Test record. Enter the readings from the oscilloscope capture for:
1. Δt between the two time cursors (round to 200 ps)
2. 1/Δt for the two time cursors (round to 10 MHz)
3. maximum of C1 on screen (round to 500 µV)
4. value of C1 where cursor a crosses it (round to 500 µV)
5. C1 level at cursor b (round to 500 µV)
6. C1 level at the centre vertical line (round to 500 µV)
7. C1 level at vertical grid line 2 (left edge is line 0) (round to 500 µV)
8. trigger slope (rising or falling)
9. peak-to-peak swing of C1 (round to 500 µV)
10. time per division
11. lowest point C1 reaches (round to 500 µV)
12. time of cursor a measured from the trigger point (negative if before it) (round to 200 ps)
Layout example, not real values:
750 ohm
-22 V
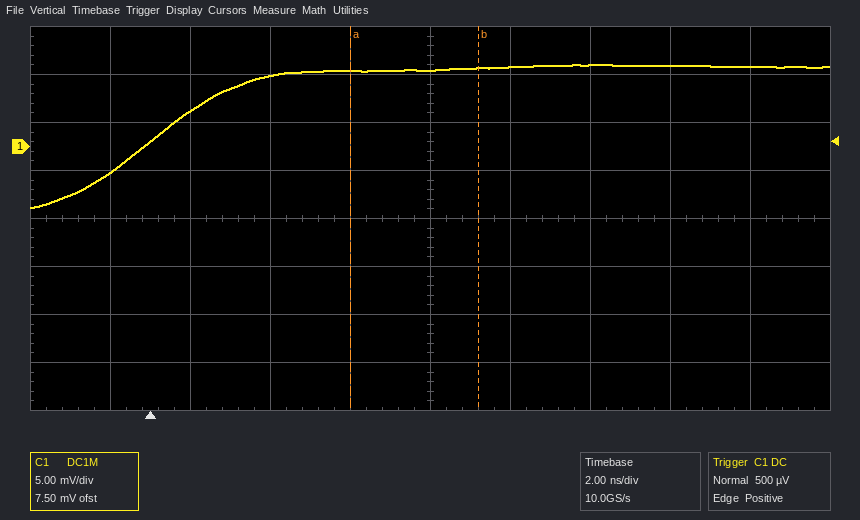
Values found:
3.2 ns
310 MHz
8.5 mV
8.0 mV
8.0 mV
8.0 mV
3.5 mV
rising
15.0 mV
2 ns
-6.5 mV
+5.0 ns
